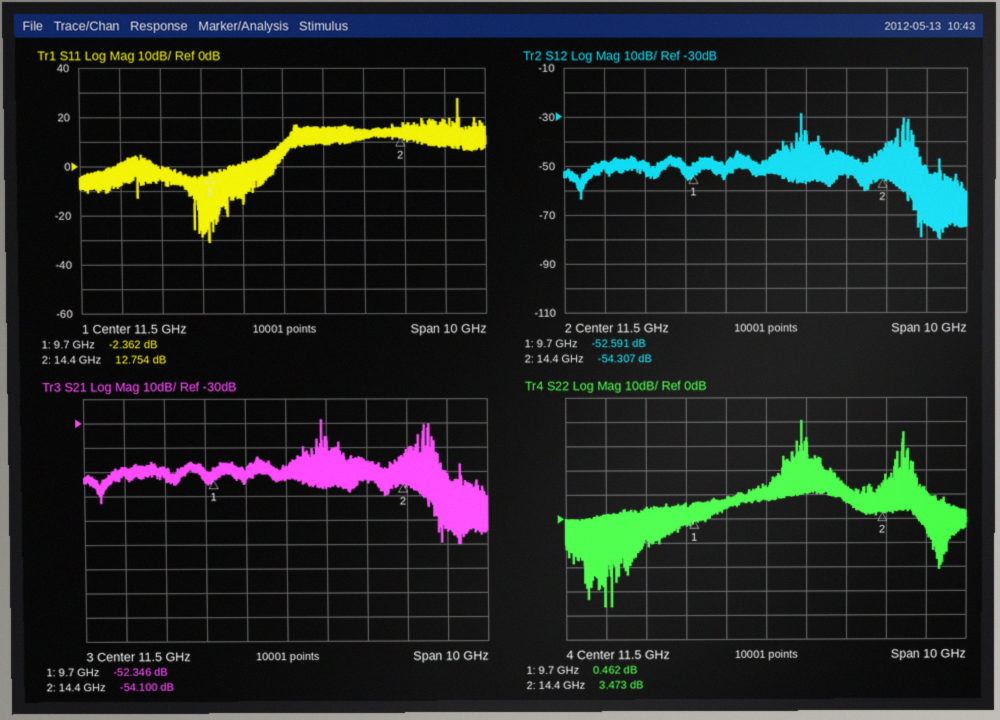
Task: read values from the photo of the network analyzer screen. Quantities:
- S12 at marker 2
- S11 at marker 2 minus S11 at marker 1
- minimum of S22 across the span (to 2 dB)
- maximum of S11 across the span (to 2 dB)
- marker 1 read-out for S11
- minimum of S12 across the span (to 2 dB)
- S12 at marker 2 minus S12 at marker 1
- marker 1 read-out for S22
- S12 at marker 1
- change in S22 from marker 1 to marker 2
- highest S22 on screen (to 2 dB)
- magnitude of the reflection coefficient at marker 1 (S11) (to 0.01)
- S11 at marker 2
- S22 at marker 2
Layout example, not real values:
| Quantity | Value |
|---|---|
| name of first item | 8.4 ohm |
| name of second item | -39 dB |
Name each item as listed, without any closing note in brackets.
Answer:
| Quantity | Value |
|---|---|
| S12 at marker 2 | -54.307 dB |
| S11 at marker 2 minus S11 at marker 1 | 15.116 dB |
| minimum of S22 across the span | -36 dB |
| maximum of S11 across the span | 28 dB |
| marker 1 read-out for S11 | -2.362 dB |
| minimum of S12 across the span | -80 dB |
| S12 at marker 2 minus S12 at marker 1 | -1.716 dB |
| marker 1 read-out for S22 | 0.462 dB |
| S12 at marker 1 | -52.591 dB |
| change in S22 from marker 1 to marker 2 | 3.011 dB |
| highest S22 on screen | 40 dB |
| magnitude of the reflection coefficient at marker 1 (S11) | 0.76 |
| S11 at marker 2 | 12.754 dB |
| S22 at marker 2 | 3.473 dB |
